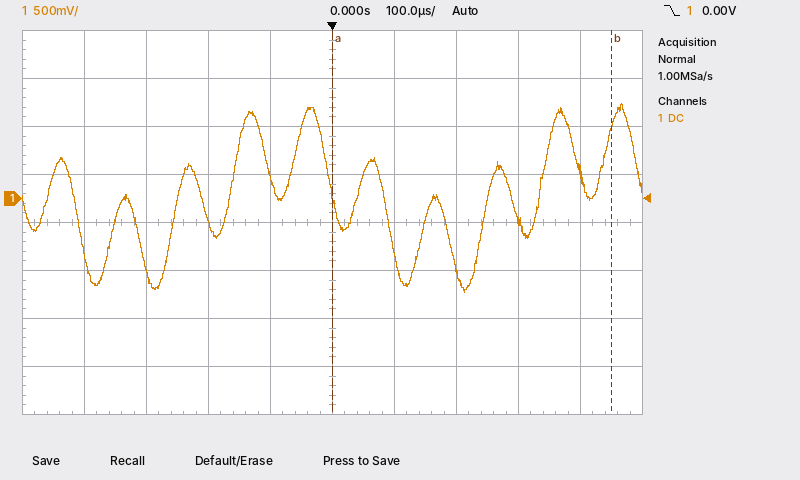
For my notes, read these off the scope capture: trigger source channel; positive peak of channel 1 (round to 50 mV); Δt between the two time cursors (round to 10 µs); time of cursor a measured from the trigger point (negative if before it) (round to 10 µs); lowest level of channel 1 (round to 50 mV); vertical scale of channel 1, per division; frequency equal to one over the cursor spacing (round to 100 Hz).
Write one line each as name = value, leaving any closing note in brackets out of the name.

trigger source channel = channel 1
positive peak of channel 1 = 1.00 V
Δt between the two time cursors = 450 µs
time of cursor a measured from the trigger point (negative if before it) = 0 µs
lowest level of channel 1 = -1.00 V
vertical scale of channel 1, per division = 500 mV
frequency equal to one over the cursor spacing = 2.2 kHz
